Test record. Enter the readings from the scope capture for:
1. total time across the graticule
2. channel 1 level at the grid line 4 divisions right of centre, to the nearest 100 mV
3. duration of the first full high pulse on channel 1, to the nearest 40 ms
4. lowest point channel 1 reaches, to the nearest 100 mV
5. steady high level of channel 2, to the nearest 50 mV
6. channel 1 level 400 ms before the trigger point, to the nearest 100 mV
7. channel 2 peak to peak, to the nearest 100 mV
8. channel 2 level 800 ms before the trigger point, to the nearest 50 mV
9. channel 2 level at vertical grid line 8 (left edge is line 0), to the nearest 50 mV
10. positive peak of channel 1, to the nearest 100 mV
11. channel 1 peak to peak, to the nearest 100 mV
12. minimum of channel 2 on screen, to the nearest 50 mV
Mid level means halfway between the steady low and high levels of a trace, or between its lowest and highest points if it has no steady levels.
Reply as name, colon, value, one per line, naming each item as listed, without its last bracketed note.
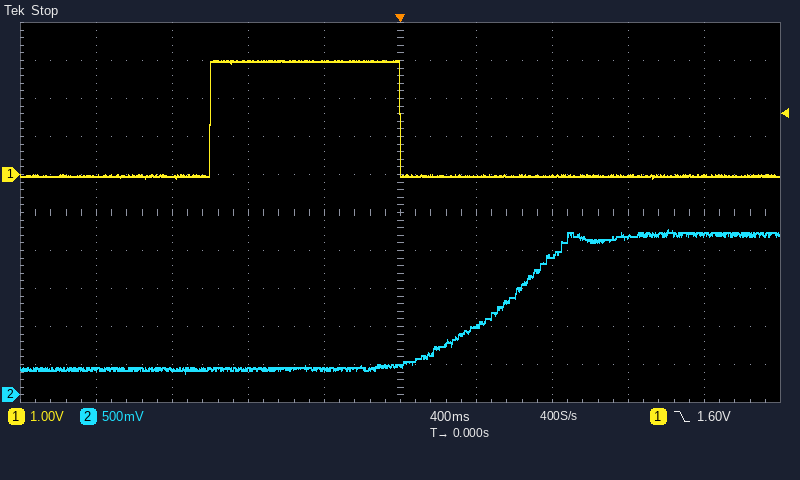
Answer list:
total time across the graticule: 4 s
channel 1 level at the grid line 4 divisions right of centre, to the nearest 100 mV: 0.0 V
duration of the first full high pulse on channel 1, to the nearest 40 ms: 1.00 s
lowest point channel 1 reaches, to the nearest 100 mV: -100 mV
steady high level of channel 2, to the nearest 50 mV: 2.10 V
channel 1 level 400 ms before the trigger point, to the nearest 100 mV: 3.0 V
channel 2 peak to peak, to the nearest 100 mV: 1.90 V
channel 2 level 800 ms before the trigger point, to the nearest 50 mV: 350 mV
channel 2 level at vertical grid line 8 (left edge is line 0), to the nearest 50 mV: 2.10 V
positive peak of channel 1, to the nearest 100 mV: 3.0 V
channel 1 peak to peak, to the nearest 100 mV: 3.1 V
minimum of channel 2 on screen, to the nearest 50 mV: 300 mV
